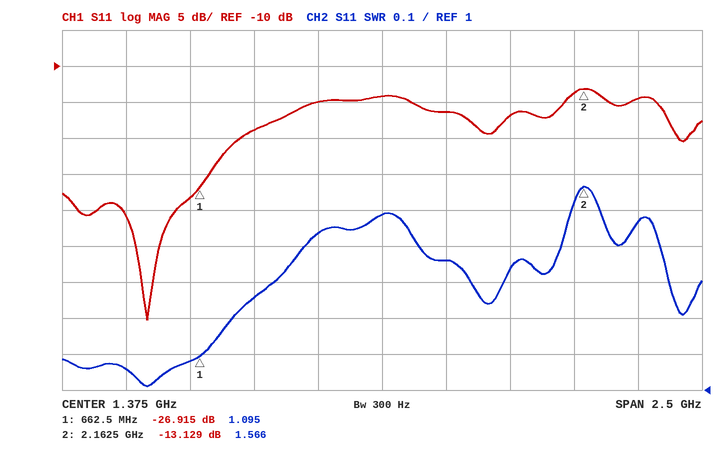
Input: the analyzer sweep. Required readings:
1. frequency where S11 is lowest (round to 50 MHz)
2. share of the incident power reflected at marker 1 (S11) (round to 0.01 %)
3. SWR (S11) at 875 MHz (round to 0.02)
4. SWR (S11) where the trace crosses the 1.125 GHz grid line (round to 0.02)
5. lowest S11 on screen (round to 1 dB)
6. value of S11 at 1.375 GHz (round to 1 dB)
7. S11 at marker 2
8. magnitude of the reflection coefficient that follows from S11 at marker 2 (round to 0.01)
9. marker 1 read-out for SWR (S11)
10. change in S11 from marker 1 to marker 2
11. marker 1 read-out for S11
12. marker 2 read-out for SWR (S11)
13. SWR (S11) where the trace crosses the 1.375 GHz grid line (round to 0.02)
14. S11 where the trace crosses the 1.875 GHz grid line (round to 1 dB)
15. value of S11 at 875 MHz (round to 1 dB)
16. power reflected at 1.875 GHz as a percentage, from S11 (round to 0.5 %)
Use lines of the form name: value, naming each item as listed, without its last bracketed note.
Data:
frequency where S11 is lowest: 450 MHz
share of the incident power reflected at marker 1 (S11): 0.20 %
SWR (S11) at 875 MHz: 1.26
SWR (S11) where the trace crosses the 1.125 GHz grid line: 1.44
lowest S11 on screen: -45 dB
value of S11 at 1.375 GHz: -14 dB
S11 at marker 2: -13.129 dB
magnitude of the reflection coefficient that follows from S11 at marker 2: 0.22
marker 1 read-out for SWR: 1.095
change in S11 from marker 1 to marker 2: 13.786 dB
marker 1 read-out for S11: -26.915 dB
marker 2 read-out for SWR: 1.566
SWR (S11) where the trace crosses the 1.375 GHz grid line: 1.48
S11 where the trace crosses the 1.875 GHz grid line: -17 dB
value of S11 at 875 MHz: -19 dB
power reflected at 1.875 GHz as a percentage, from S11: 2.0 %
